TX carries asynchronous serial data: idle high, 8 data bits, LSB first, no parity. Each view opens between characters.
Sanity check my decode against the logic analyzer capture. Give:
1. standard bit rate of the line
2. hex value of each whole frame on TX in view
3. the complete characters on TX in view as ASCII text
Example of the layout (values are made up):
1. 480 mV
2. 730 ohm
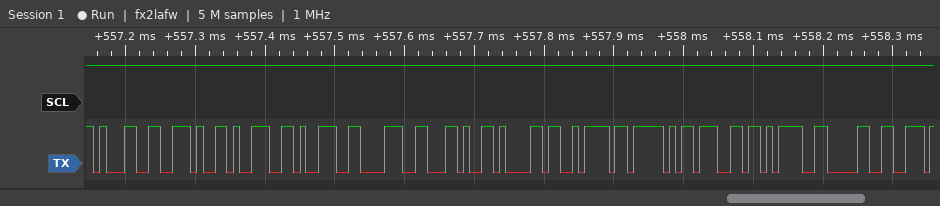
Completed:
1. 115200 baud
2. 31, 2E, 39, 39, 38, 2C, 61, 7A, 5F, 67, 3D, 30
3. "1.998,az_g=0"
